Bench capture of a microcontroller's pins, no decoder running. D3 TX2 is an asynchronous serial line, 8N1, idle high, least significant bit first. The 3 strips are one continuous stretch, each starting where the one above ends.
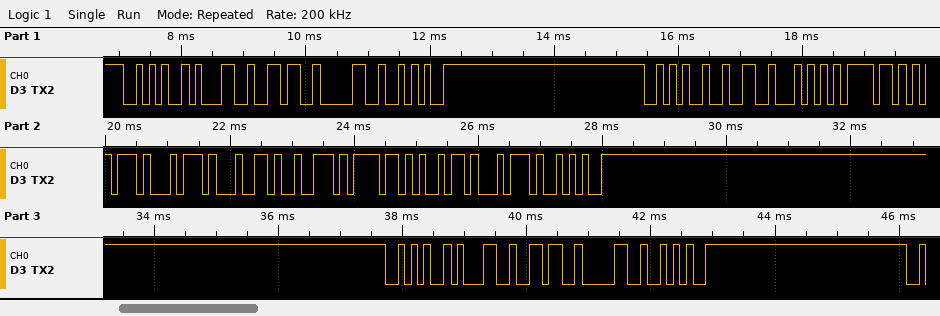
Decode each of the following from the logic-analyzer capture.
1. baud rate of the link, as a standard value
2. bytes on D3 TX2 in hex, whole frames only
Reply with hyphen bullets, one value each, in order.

- 9600 baud
- 2A 31 36 30 2A 2A 32 54 6F 75 74 64 72 6F 69 74 2A 2A 31 36 30 2A
